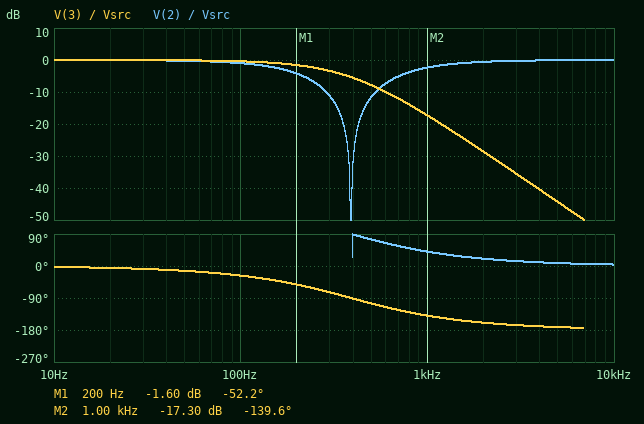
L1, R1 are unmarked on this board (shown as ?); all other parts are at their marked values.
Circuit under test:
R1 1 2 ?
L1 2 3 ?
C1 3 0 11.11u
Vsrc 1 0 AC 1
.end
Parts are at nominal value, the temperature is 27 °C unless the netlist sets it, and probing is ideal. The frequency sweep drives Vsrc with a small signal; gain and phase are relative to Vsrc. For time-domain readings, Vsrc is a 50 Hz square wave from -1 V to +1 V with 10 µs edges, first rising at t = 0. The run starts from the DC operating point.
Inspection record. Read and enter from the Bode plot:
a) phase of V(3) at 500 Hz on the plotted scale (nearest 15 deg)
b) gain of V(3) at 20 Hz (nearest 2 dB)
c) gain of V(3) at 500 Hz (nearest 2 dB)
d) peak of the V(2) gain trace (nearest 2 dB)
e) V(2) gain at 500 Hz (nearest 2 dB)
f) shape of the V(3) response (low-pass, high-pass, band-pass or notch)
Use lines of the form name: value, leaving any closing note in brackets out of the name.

phase of V(3) at 500 Hz on the plotted scale: -105 deg
gain of V(3) at 20 Hz: 0 dB
gain of V(3) at 500 Hz: -8 dB
peak of the V(2) gain trace: 0 dB
V(2) gain at 500 Hz: -12 dB
shape of the V(3) response: low-pass
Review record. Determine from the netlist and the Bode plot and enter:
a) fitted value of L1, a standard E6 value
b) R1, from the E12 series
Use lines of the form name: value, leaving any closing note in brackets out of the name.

fitted value of L1, a standard E6 value: 15 mH
R1, from the E12 series: 68 Ω
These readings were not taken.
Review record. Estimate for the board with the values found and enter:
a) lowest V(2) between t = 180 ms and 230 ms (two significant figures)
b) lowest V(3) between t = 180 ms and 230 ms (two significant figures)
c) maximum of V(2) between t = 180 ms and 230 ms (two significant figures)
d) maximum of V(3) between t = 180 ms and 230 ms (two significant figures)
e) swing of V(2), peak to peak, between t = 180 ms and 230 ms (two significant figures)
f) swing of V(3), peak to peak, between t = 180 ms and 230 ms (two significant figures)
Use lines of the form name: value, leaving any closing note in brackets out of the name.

lowest V(2) between t = 180 ms and 230 ms: -1.0 V
lowest V(3) between t = 180 ms and 230 ms: -1.0 V
maximum of V(2) between t = 180 ms and 230 ms: 1.0 V
maximum of V(3) between t = 180 ms and 230 ms: 1.0 V
swing of V(2), peak to peak, between t = 180 ms and 230 ms: 2.0 V
swing of V(3), peak to peak, between t = 180 ms and 230 ms: 2.0 V
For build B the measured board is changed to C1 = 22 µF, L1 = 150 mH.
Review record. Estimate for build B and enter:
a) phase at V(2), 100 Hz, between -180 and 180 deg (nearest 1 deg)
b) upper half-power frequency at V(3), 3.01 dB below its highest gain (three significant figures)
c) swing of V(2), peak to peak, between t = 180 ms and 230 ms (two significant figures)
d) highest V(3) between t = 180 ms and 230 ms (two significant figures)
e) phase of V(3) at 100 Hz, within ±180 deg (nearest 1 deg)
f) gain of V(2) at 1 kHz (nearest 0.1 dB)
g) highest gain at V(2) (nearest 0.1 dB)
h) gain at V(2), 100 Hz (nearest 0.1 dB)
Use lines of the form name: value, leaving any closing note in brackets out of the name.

phase at V(2), 100 Hz, between -180 and 180 deg: 72 deg
upper half-power frequency at V(3), 3.01 dB below its highest gain: 104 Hz
swing of V(2), peak to peak, between t = 180 ms and 230 ms: 2.5 V
highest V(3) between t = 180 ms and 230 ms: 1.5 V
phase of V(3) at 100 Hz, within ±180 deg: -108 deg
gain of V(2) at 1 kHz: 0 dB
highest gain at V(2): 0 dB
gain at V(2), 100 Hz: -10.3 dB
